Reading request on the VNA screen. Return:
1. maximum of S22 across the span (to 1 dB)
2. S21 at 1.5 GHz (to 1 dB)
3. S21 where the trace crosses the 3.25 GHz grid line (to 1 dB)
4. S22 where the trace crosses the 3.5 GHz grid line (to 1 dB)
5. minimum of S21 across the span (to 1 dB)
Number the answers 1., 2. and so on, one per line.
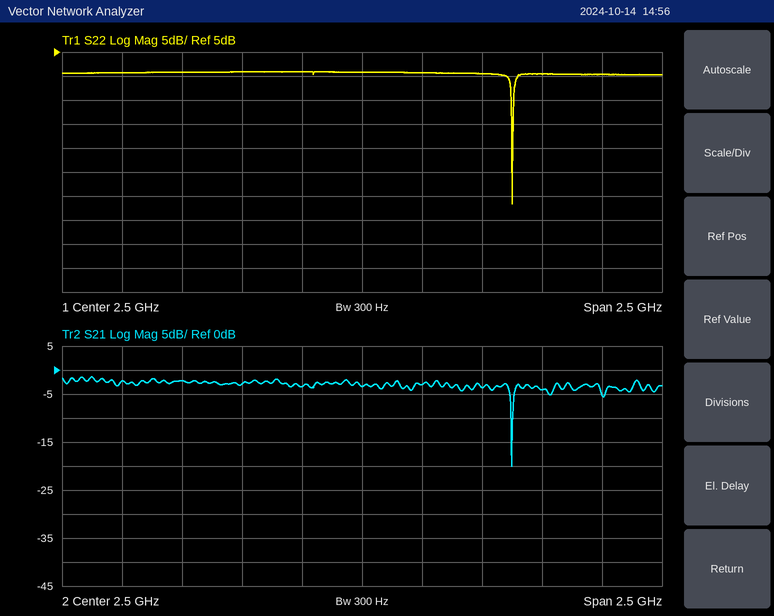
1. 1 dB
2. -2 dB
3. -4 dB
4. 0 dB
5. -20 dB
